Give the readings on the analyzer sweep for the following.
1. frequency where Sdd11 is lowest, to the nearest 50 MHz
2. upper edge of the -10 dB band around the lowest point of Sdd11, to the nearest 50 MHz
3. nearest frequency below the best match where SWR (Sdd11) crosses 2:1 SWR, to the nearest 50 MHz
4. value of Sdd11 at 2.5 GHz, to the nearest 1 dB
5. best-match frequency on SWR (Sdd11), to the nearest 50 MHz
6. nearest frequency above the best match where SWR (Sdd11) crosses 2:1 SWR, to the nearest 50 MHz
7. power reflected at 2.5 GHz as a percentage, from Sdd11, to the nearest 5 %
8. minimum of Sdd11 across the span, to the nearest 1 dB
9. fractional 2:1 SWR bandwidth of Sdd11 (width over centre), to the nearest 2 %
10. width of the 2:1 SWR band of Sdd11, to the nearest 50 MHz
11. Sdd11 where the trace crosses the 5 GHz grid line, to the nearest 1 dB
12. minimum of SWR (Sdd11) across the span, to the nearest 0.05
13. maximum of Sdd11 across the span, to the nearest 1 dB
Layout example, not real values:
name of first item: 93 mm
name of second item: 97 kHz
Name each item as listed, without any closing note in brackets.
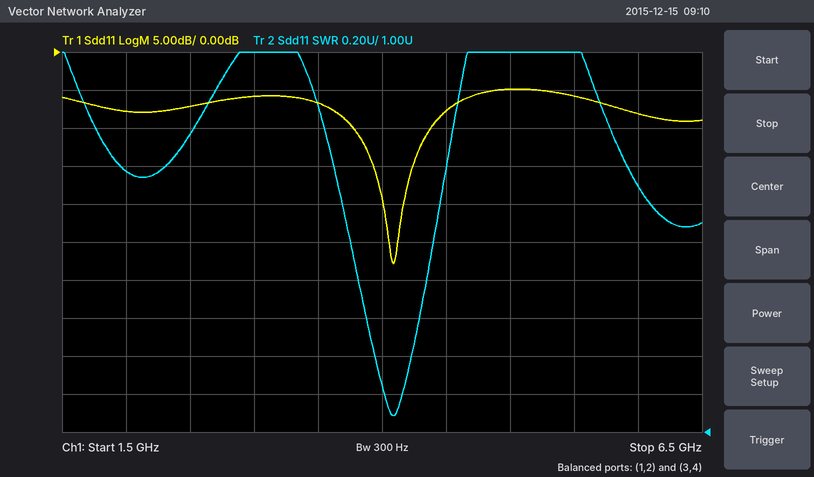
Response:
frequency where Sdd11 is lowest, to the nearest 50 MHz: 4.10 GHz
upper edge of the -10 dB band around the lowest point of Sdd11, to the nearest 50 MHz: 4.40 GHz
nearest frequency below the best match where SWR (Sdd11) crosses 2:1 SWR, to the nearest 50 MHz: 3.75 GHz
value of Sdd11 at 2.5 GHz, to the nearest 1 dB: -7 dB
best-match frequency on SWR (Sdd11), to the nearest 50 MHz: 4.10 GHz
nearest frequency above the best match where SWR (Sdd11) crosses 2:1 SWR, to the nearest 50 MHz: 4.40 GHz
power reflected at 2.5 GHz as a percentage, from Sdd11, to the nearest 5 %: 20 %
minimum of Sdd11 across the span, to the nearest 1 dB: -28 dB
fractional 2:1 SWR bandwidth of Sdd11 (width over centre), to the nearest 2 %: 16 %
width of the 2:1 SWR band of Sdd11, to the nearest 50 MHz: 650 MHz
Sdd11 where the trace crosses the 5 GHz grid line, to the nearest 1 dB: -5 dB
minimum of SWR (Sdd11) across the span, to the nearest 0.05: 1.10
maximum of Sdd11 across the span, to the nearest 1 dB: -5 dB
